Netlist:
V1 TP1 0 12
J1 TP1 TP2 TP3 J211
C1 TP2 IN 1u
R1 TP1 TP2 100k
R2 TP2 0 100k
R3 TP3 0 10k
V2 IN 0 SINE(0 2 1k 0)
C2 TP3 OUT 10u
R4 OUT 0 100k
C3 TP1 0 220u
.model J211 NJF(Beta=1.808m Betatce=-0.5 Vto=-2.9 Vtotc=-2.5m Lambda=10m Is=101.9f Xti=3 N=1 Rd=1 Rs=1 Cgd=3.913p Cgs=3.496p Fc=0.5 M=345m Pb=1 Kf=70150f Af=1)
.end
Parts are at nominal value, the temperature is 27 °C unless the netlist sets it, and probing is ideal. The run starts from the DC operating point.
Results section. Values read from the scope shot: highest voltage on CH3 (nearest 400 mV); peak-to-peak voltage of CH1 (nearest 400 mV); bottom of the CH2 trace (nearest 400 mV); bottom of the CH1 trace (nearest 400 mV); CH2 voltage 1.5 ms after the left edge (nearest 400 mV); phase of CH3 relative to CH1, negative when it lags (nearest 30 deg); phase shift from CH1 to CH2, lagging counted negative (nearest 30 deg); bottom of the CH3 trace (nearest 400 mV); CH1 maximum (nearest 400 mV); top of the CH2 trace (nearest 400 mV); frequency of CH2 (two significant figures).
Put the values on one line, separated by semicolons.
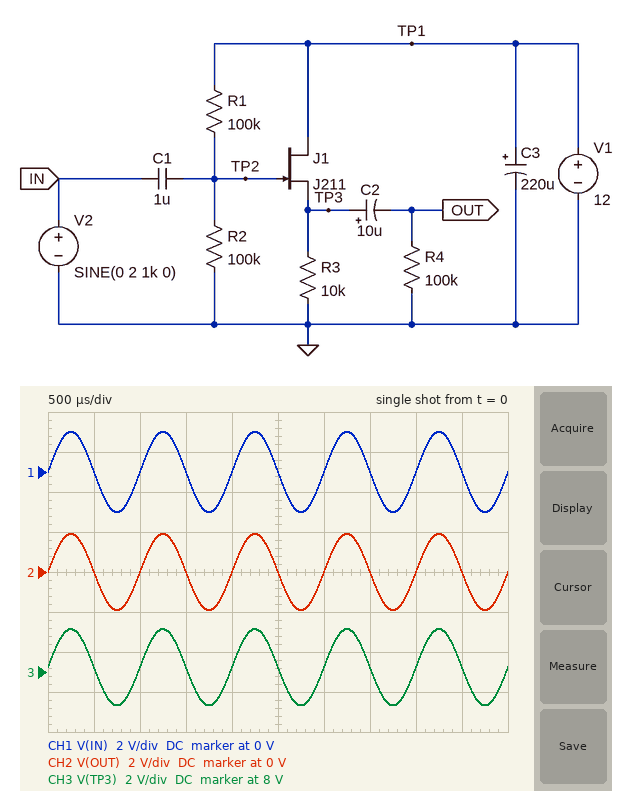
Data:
10.0 V; 4.0 V; -2.0 V; -2.0 V; 0 V; 0 deg; 0 deg; 6.4 V; 2.0 V; 2.0 V; 1.0 kHz
